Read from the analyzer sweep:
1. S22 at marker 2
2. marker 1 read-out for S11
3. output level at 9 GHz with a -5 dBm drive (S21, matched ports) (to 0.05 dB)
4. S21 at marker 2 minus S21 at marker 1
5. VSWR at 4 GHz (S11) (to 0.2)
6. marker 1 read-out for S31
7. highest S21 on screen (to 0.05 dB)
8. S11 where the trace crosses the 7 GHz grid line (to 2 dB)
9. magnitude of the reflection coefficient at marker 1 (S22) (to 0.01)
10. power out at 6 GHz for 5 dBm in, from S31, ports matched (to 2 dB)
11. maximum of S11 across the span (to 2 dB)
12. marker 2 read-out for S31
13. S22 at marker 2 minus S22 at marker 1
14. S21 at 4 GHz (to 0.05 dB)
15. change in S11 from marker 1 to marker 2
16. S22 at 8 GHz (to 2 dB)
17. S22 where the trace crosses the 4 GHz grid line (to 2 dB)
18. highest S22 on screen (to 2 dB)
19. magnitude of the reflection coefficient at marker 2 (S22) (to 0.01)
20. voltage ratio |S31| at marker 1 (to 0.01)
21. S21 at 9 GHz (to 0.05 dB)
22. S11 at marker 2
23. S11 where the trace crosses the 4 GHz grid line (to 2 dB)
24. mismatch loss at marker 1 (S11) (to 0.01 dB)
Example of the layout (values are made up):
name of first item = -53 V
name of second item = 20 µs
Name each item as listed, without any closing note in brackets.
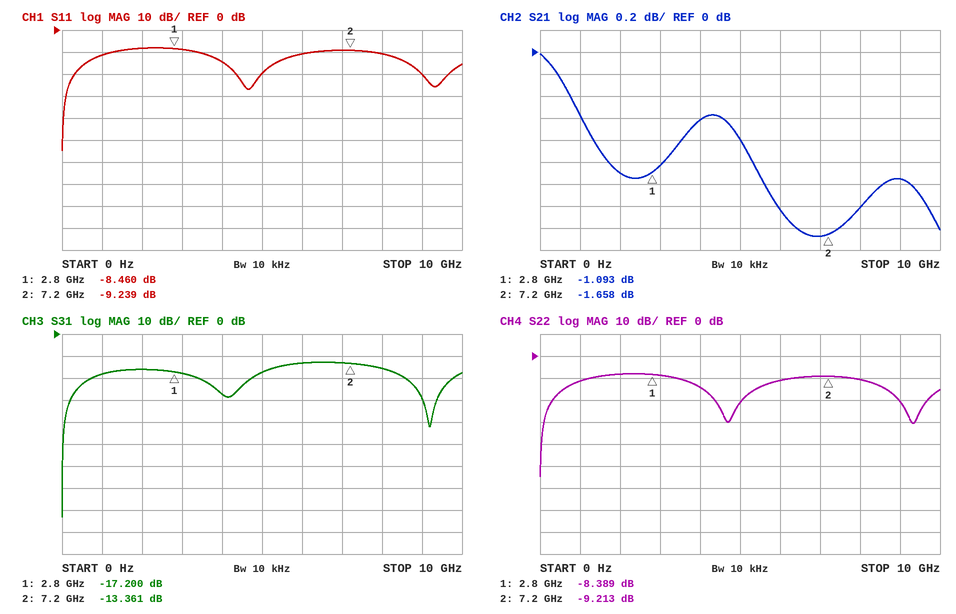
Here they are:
S22 at marker 2 = -9.213 dB
marker 1 read-out for S11 = -8.460 dB
output level at 9 GHz with a -5 dBm drive (S21, matched ports) = -6.15 dBm
S21 at marker 2 minus S21 at marker 1 = -0.565 dB
VSWR at 4 GHz (S11) = 1.4
marker 1 read-out for S31 = -17.200 dB
highest S21 on screen = 0.00 dB
S11 where the trace crosses the 7 GHz grid line = -10 dB
magnitude of the reflection coefficient at marker 1 (S22) = 0.38
power out at 6 GHz for 5 dBm in, from S31, ports matched = -8 dBm
maximum of S11 across the span = -8 dB
marker 2 read-out for S31 = -13.361 dB
S22 at marker 2 minus S22 at marker 1 = -0.824 dB
S21 at 4 GHz = -0.60 dB
change in S11 from marker 1 to marker 2 = -0.779 dB
S22 at 8 GHz = -10 dB
S22 where the trace crosses the 4 GHz grid line = -14 dB
highest S22 on screen = -8 dB
magnitude of the reflection coefficient at marker 2 (S22) = 0.35
voltage ratio |S31| at marker 1 = 0.14
S21 at 9 GHz = -1.15 dB
S11 at marker 2 = -9.239 dB
S11 where the trace crosses the 4 GHz grid line = -14 dB
mismatch loss at marker 1 (S11) = 0.67 dB
